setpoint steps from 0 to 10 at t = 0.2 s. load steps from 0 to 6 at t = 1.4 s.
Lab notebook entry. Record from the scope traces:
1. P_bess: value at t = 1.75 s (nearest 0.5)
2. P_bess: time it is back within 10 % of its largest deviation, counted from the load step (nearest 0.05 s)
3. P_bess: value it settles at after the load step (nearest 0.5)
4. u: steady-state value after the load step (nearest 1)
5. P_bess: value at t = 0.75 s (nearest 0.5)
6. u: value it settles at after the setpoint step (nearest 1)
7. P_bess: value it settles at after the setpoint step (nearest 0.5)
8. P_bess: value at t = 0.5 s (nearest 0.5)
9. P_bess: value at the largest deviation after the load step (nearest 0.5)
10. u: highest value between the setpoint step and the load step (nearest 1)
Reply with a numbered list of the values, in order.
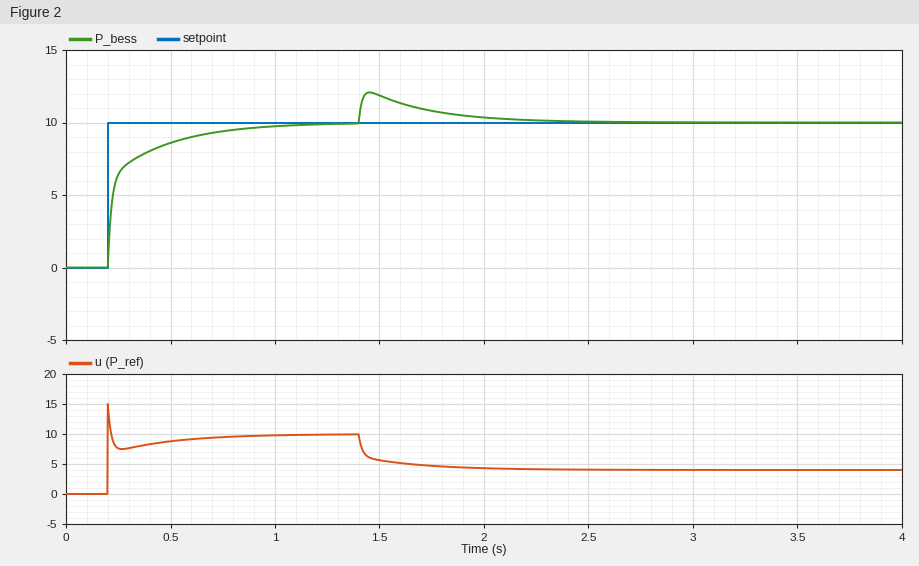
1. 11.0
2. 0.75 s
3. 10.0
4. 4
5. 9.5
6. 10
7. 10.0
8. 8.5
9. 12.0
10. 15
